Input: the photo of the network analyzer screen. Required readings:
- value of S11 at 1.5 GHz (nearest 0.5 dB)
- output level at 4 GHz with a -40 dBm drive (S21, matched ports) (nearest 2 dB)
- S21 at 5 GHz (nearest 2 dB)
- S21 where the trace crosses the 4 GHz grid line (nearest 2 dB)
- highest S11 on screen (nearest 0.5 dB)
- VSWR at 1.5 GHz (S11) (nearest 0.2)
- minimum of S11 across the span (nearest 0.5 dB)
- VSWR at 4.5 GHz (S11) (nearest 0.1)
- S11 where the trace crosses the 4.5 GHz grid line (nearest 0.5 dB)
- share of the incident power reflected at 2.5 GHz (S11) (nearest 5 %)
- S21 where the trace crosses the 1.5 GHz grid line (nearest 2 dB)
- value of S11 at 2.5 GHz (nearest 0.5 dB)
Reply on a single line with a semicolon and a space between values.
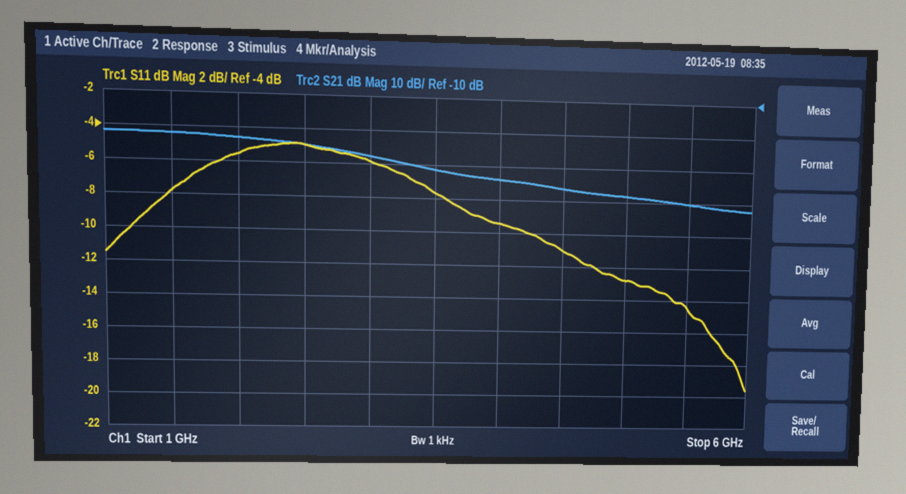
-8.0 dB; -74 dBm; -38 dB; -34 dB; -5.0 dB; 2.4; -19.5 dB; 1.8; -11.0 dB; 30 %; -22 dB; -5.0 dB
